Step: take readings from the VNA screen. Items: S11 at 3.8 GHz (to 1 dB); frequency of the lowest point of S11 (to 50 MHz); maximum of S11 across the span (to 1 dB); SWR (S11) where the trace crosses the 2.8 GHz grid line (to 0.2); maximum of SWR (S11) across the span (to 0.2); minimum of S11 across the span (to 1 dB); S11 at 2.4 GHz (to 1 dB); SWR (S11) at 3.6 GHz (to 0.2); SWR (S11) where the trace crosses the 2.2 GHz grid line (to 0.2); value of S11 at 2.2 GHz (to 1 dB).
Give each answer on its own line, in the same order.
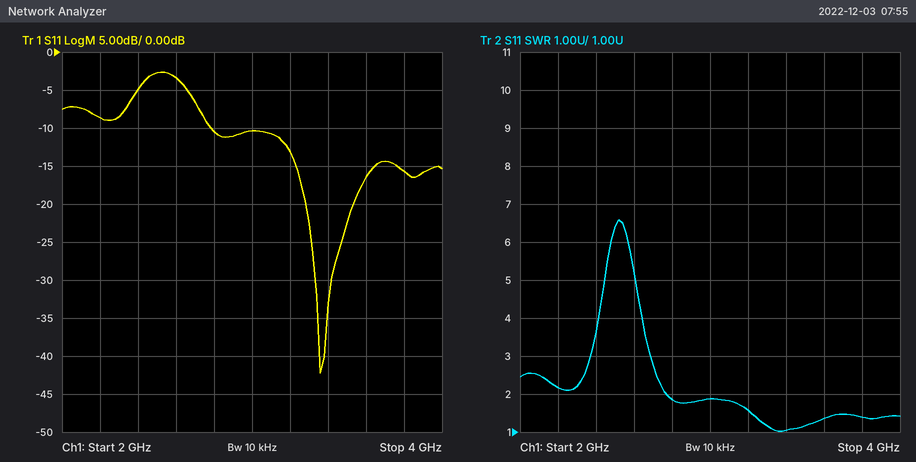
-16 dB
3.35 GHz
-3 dB
1.8
6.6
-42 dB
-5 dB
1.4
2.2
-9 dB
